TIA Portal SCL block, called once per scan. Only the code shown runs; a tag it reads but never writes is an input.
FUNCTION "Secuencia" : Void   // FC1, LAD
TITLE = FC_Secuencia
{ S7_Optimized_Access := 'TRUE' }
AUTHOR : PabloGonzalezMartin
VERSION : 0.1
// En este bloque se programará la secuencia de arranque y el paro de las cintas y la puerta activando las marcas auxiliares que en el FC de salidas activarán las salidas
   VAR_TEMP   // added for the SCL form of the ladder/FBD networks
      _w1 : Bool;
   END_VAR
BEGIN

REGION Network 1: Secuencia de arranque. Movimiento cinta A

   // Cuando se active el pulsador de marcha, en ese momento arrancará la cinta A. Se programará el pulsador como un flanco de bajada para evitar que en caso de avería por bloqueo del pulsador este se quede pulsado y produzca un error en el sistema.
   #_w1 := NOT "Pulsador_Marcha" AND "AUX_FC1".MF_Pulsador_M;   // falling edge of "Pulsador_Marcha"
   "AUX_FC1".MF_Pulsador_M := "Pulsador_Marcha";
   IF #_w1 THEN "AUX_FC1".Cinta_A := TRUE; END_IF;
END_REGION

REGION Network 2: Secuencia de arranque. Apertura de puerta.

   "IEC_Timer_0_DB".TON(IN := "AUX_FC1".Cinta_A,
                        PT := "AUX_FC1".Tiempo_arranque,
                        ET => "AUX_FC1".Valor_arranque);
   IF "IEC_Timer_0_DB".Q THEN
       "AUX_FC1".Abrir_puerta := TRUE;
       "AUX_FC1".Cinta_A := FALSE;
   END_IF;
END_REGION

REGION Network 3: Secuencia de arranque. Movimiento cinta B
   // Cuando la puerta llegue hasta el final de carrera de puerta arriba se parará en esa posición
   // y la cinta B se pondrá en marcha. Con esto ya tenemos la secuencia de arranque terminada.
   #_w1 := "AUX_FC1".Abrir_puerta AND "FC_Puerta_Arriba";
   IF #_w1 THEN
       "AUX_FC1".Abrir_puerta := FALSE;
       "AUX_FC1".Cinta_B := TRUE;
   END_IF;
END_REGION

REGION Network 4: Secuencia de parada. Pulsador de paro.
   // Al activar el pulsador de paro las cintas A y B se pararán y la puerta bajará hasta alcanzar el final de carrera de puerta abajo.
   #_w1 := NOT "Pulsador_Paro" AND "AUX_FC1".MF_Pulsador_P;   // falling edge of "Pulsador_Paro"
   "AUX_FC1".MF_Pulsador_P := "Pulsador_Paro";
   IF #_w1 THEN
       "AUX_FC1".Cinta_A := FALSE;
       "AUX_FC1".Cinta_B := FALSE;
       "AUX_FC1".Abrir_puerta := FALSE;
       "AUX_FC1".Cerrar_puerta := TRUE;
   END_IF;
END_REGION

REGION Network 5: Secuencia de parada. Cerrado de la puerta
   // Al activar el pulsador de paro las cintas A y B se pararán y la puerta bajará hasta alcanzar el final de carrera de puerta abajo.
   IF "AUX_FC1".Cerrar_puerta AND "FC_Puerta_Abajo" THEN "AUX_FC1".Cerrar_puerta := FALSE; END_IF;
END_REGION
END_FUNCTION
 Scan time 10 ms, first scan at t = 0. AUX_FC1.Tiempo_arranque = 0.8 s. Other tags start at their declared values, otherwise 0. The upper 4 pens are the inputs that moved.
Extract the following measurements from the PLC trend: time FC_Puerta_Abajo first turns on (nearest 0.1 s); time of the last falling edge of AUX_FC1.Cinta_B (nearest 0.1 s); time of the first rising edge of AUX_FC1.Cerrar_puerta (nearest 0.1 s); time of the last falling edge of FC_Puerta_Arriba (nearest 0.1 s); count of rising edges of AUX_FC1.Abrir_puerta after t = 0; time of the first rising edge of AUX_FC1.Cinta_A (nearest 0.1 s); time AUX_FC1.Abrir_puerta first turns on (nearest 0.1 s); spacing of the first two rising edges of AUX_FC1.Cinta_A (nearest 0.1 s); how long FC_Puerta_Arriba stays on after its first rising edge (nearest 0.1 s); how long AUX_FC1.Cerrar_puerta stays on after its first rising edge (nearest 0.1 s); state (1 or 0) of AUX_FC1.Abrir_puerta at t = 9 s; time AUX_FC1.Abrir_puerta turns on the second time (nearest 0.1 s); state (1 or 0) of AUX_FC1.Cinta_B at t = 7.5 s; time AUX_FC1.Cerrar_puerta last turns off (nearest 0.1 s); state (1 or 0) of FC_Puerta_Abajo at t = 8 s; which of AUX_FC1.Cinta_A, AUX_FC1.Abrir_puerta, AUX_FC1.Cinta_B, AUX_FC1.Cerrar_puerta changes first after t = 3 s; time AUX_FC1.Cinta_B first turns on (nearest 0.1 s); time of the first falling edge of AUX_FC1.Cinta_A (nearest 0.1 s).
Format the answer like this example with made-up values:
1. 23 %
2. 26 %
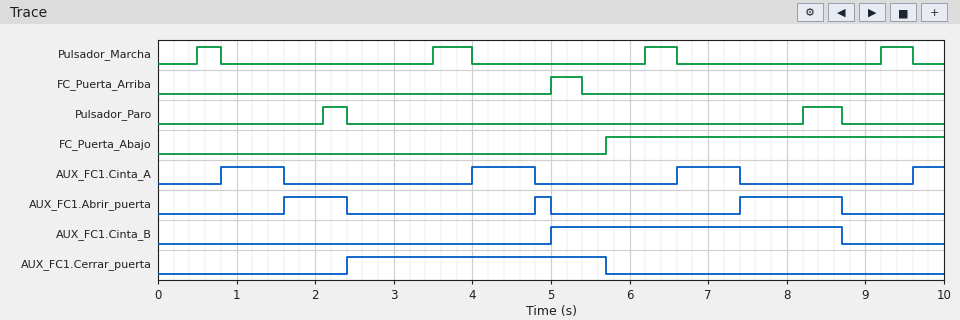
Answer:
1. 5.7 s
2. 8.7 s
3. 2.4 s
4. 5.4 s
5. 3
6. 0.8 s
7. 1.6 s
8. 3.2 s
9. 0.4 s
10. 3.3 s
11. 0
12. 4.8 s
13. 1
14. 5.7 s
15. 1
16. AUX_FC1.Cinta_A
17. 5.0 s
18. 1.6 s
